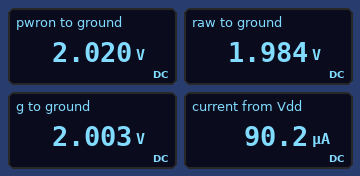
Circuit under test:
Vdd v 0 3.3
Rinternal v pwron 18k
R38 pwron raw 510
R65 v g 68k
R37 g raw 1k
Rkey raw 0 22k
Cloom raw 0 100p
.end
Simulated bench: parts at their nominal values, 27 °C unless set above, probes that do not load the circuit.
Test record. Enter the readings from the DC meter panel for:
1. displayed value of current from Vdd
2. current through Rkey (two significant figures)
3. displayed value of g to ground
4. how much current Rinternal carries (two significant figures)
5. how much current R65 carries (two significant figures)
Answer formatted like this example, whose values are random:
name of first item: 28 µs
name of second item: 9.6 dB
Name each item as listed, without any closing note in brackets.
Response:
displayed value of current from Vdd: 90.2 µA
current through Rkey: 90 µA
displayed value of g to ground: 2.003 V
how much current Rinternal carries: 71 µA
how much current R65 carries: 19 µA
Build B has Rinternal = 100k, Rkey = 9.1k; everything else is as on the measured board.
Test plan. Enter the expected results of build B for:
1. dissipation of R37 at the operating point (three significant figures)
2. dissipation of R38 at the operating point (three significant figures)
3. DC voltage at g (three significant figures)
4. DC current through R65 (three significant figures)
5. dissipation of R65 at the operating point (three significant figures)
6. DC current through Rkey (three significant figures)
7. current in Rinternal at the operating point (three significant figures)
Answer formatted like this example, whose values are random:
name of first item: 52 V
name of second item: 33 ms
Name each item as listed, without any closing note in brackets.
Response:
dissipation of R37 at the operating point: 1.53 µW
dissipation of R38 at the operating point: 368 nW
DC voltage at g: 640 mV
DC current through R65: 39.1 µA
dissipation of R65 at the operating point: 104 µW
DC current through Rkey: 66.0 µA
current in Rinternal at the operating point: 26.9 µA
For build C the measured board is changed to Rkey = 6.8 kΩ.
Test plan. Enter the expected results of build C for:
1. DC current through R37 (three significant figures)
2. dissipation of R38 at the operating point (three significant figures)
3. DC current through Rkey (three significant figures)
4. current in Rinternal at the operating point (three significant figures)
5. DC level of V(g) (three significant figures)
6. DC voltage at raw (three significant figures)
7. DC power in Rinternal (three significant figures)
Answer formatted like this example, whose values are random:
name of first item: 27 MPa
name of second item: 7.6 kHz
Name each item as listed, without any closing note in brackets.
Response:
DC current through R37: 32.6 µA
dissipation of R38 at the operating point: 7.54 µW
DC current through Rkey: 154 µA
current in Rinternal at the operating point: 122 µA
DC level of V(g): 1.08 V
DC voltage at raw: 1.05 V
DC power in Rinternal: 266 µW
